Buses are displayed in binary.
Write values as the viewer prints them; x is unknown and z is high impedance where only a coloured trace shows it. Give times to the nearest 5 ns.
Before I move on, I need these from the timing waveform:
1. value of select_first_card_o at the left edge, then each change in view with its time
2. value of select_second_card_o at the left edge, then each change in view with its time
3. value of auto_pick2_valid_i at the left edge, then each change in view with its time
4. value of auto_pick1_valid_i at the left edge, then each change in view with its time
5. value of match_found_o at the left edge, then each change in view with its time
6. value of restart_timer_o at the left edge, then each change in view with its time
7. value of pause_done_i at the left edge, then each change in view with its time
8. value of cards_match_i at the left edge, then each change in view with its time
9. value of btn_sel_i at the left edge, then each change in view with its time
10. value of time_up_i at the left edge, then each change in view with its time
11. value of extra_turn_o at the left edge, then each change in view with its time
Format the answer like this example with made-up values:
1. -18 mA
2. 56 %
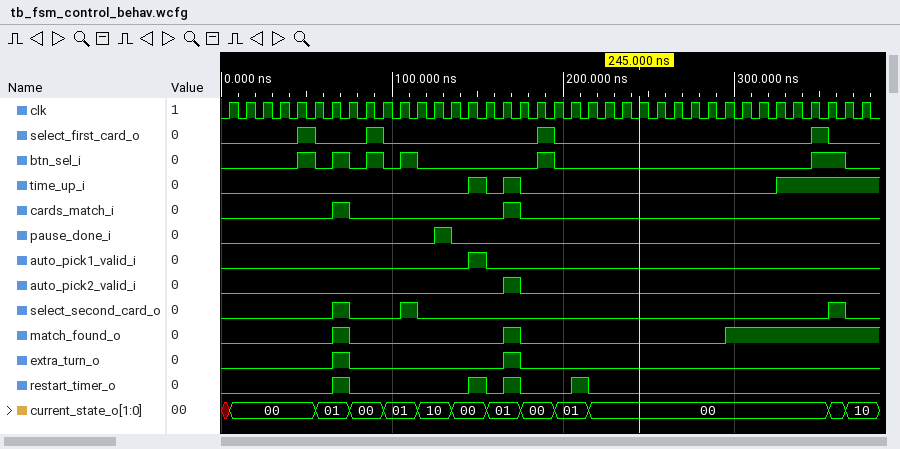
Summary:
1. 0, 1 at 45 ns, 0 at 55 ns, 1 at 85 ns, 0 at 95 ns, 1 at 185 ns, 0 at 195 ns, 1 at 345 ns, 0 at 355 ns
2. 0, 1 at 65 ns, 0 at 75 ns, 1 at 105 ns, 0 at 115 ns, 1 at 355 ns, 0 at 365 ns
3. 0, 1 at 165 ns, 0 at 175 ns
4. 0, 1 at 145 ns, 0 at 155 ns
5. 0, 1 at 65 ns, 0 at 75 ns, 1 at 165 ns, 0 at 175 ns, 1 at 295 ns
6. 0, 1 at 65 ns, 0 at 75 ns, 1 at 145 ns, 0 at 155 ns, 1 at 165 ns, 0 at 175 ns, 1 at 205 ns, 0 at 215 ns
7. 0, 1 at 125 ns, 0 at 135 ns
8. 0, 1 at 65 ns, 0 at 75 ns, 1 at 165 ns, 0 at 175 ns
9. 0, 1 at 45 ns, 0 at 55 ns, 1 at 65 ns, 0 at 75 ns, 1 at 85 ns, 0 at 95 ns, 1 at 105 ns, 0 at 115 ns, 1 at 185 ns, 0 at 195 ns, 1 at 345 ns, 0 at 365 ns
10. 0, 1 at 145 ns, 0 at 155 ns, 1 at 165 ns, 0 at 175 ns, 1 at 325 ns
11. 0, 1 at 65 ns, 0 at 75 ns, 1 at 165 ns, 0 at 175 ns
